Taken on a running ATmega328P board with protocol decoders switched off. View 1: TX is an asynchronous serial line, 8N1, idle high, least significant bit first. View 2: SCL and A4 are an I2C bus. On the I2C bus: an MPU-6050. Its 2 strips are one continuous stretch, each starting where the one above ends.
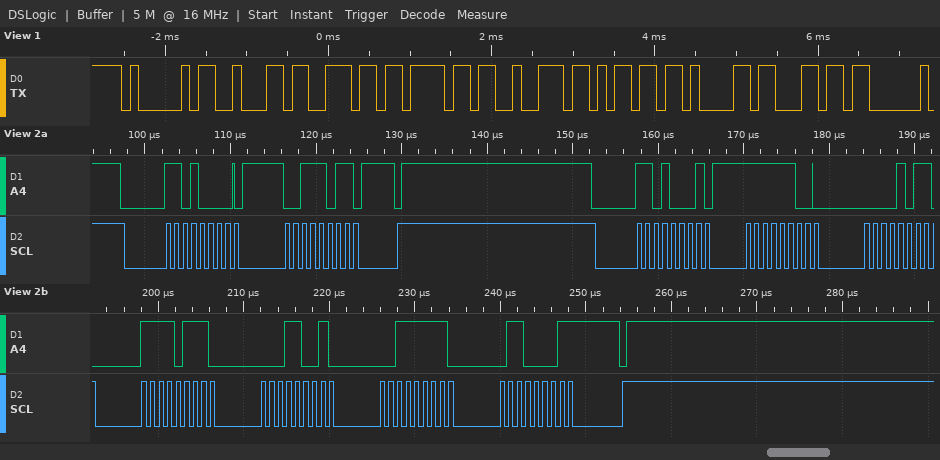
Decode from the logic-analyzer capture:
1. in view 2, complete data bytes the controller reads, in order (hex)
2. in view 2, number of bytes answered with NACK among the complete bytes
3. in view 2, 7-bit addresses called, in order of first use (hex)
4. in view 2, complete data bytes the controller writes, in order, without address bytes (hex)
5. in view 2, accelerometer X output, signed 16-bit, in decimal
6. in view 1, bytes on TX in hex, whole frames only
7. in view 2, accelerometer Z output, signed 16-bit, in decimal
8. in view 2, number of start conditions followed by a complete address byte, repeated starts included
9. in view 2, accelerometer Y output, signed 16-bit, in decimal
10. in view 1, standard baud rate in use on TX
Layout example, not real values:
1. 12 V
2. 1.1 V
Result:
1. FC 0B F7 19 3F 61
2. 1
3. 0x68
4. 3B
5. -1013
6. 0x41 0x62 0x6E 0x6F 0x72 0x6D 0x61 0x6C
7. 16225
8. 2
9. -2279
10. 9600 baud
